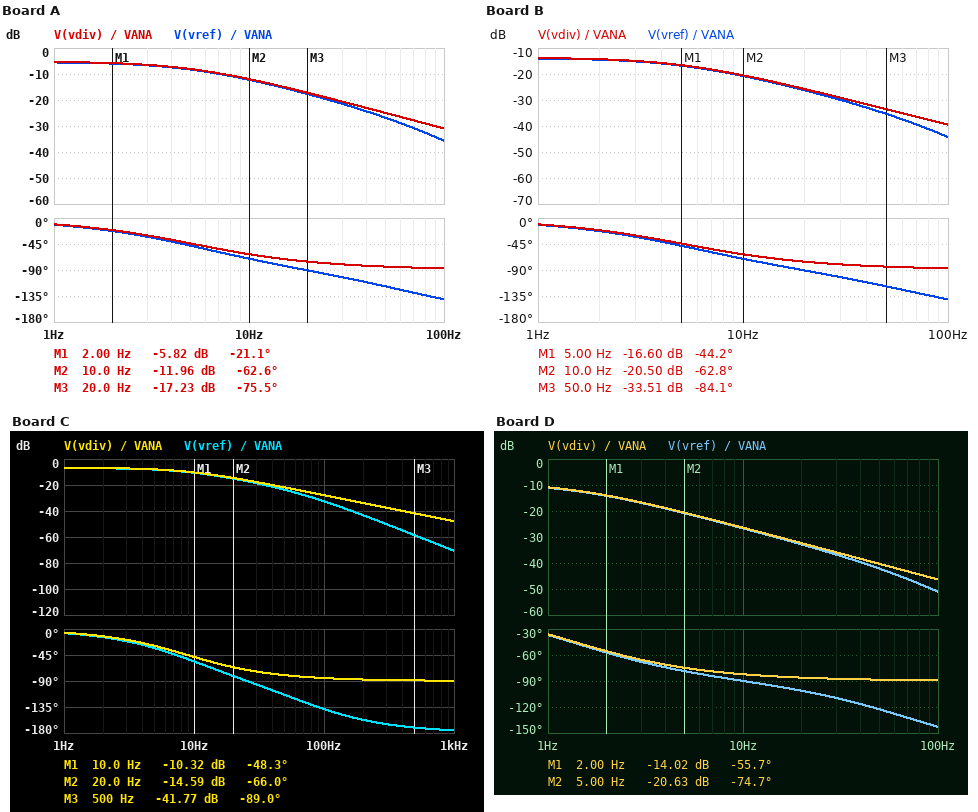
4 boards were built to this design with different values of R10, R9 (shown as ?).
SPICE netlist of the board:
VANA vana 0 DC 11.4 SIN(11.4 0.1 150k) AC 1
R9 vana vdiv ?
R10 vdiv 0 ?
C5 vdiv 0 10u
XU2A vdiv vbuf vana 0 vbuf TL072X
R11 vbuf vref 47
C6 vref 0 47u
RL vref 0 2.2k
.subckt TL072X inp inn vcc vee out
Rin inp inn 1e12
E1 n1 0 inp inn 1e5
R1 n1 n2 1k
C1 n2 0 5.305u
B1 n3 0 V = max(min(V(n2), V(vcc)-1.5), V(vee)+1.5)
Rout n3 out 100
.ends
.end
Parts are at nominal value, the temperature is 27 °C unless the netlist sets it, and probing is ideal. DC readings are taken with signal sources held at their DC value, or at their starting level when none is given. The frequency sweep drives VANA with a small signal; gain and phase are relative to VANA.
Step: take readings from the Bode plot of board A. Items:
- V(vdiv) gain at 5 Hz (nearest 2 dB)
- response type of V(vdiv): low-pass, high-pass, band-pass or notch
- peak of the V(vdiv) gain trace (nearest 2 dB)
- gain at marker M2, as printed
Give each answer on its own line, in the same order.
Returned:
-8 dB
low-pass
-6 dB
-11.96 dB
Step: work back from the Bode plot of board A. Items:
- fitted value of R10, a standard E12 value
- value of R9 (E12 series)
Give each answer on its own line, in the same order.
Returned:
6.8 kΩ
5.6 kΩ
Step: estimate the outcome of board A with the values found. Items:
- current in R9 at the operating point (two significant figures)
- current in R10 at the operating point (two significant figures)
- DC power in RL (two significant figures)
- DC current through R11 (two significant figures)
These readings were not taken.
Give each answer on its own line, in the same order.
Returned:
920 µA
920 µA
17 mW
2.8 mA
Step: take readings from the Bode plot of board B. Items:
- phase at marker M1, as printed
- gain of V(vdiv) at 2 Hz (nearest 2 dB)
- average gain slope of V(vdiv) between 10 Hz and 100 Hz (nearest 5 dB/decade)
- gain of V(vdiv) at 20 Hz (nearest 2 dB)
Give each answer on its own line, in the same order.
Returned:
-44.2 deg
-14 dB
-20 dB/decade
-26 dB
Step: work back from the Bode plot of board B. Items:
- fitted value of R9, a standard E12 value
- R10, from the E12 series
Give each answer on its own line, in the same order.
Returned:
15 kΩ
3.9 kΩ
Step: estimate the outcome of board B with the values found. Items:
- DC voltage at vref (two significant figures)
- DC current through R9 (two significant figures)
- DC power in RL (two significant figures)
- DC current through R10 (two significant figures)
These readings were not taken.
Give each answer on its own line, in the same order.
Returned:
2.3 V
600 µA
2.4 mW
600 µA
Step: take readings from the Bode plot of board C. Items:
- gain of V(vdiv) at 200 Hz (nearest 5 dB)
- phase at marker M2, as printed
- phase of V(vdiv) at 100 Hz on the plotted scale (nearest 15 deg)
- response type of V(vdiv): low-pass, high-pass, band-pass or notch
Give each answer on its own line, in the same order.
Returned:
-35 dB
-66.0 deg
-90 deg
low-pass
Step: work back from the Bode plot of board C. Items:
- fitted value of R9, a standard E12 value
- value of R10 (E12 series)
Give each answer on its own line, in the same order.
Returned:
3.9 kΩ
3.3 kΩ
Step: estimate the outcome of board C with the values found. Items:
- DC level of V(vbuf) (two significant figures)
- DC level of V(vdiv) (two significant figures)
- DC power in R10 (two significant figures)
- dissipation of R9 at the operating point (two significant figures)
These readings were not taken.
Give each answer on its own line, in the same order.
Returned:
5.2 V
5.2 V
8.3 mW
9.8 mW
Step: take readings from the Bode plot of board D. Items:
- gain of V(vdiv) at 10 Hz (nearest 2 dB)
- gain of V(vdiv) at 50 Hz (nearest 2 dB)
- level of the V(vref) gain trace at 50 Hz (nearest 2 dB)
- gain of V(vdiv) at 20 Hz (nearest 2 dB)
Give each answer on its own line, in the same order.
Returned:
-26 dB
-40 dB
-42 dB
-32 dB
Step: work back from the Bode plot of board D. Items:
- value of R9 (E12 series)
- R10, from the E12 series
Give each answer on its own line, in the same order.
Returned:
33 kΩ
18 kΩ
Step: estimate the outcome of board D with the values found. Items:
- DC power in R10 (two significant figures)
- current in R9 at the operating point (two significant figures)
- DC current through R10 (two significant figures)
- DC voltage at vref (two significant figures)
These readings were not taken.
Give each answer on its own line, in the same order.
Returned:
900 µW
220 µA
220 µA
3.9 V
